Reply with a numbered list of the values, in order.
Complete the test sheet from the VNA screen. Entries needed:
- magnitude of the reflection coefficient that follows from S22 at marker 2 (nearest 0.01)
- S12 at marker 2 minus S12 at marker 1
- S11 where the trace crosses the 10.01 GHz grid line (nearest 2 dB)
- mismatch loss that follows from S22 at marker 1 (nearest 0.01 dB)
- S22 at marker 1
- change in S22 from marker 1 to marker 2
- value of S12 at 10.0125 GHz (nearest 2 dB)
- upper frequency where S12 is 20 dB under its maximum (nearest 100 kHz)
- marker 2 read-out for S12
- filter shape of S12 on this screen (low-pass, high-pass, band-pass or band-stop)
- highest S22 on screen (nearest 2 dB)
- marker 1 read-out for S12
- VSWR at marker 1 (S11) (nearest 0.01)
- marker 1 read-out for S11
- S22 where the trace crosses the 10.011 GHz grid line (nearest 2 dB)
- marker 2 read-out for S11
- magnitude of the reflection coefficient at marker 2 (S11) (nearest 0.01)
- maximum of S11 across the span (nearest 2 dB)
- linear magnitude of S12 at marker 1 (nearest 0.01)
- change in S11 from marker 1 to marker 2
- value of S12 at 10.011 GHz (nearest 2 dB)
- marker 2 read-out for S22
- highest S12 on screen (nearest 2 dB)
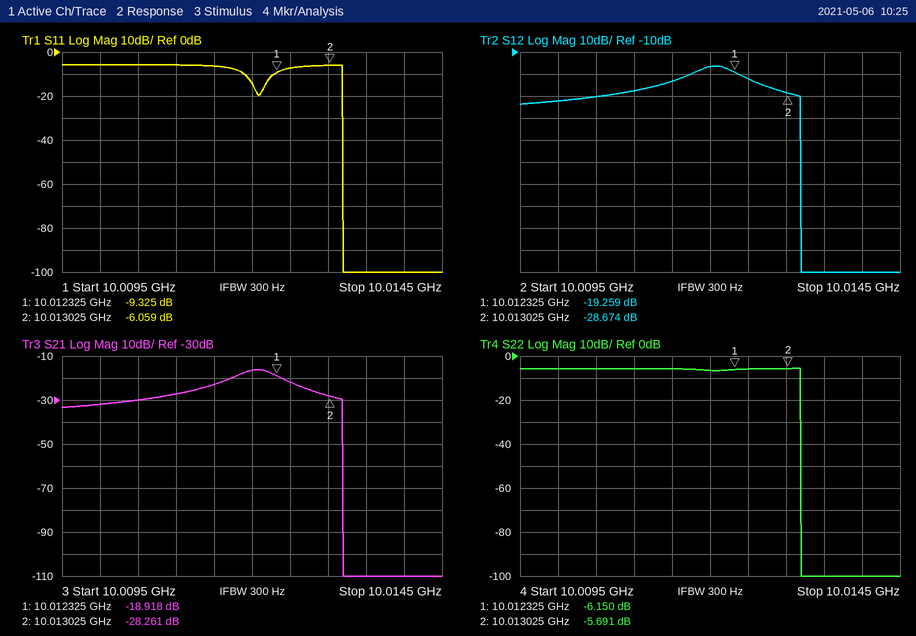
1. 0.52
2. -9.415 dB
3. -6 dB
4. 1.21 dB
5. -6.150 dB
6. 0.459 dB
7. -22 dB
8. 10.0132 GHz
9. -28.674 dB
10. band-pass
11. -6 dB
12. -19.259 dB
13. 2.04
14. -9.325 dB
15. -6 dB
16. -6.059 dB
17. 0.50
18. -6 dB
19. 0.11
20. 3.266 dB
21. -28 dB
22. -5.691 dB
23. -16 dB
